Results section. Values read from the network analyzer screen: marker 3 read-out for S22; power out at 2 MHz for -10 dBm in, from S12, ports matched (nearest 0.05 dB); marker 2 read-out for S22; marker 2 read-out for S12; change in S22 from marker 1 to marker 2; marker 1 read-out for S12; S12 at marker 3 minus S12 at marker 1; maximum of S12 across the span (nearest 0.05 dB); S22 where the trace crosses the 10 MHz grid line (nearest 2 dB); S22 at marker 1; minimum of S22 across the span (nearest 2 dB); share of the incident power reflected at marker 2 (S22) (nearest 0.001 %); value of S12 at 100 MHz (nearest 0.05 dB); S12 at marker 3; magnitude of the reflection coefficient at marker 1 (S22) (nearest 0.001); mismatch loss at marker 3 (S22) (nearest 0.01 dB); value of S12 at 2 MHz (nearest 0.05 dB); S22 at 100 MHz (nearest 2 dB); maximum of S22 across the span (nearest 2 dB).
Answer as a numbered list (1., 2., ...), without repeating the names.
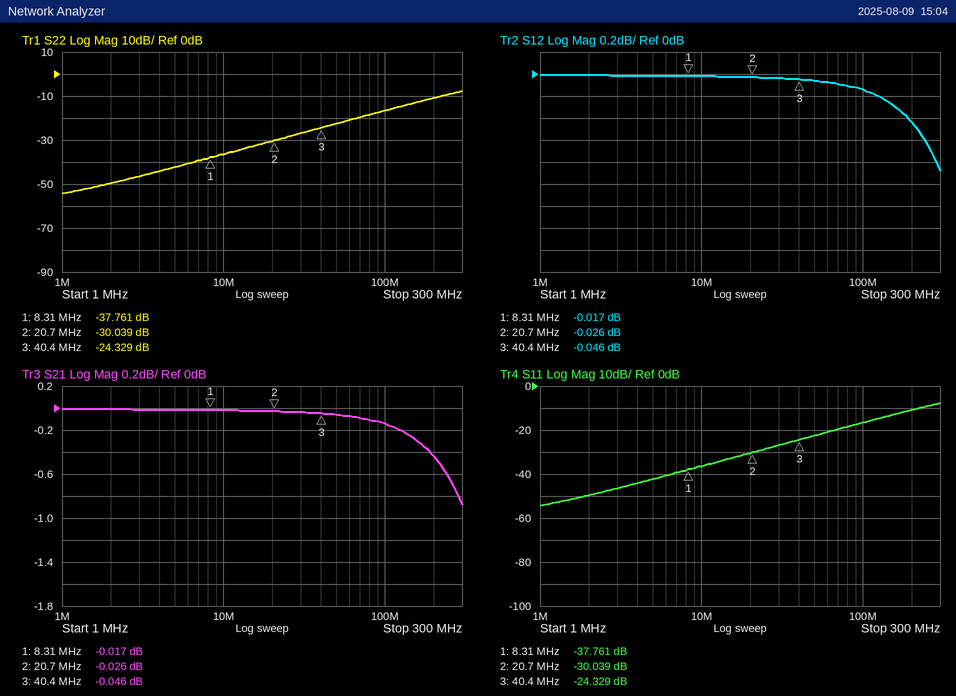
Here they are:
1. -24.329 dB
2. -10.00 dBm
3. -30.039 dB
4. -0.026 dB
5. 7.722 dB
6. -0.017 dB
7. -0.029 dB
8. 0.00 dB
9. -36 dB
10. -37.761 dB
11. -54 dB
12. 0.099 %
13. -0.15 dB
14. -0.046 dB
15. 0.013
16. 0.02 dB
17. 0.00 dB
18. -16 dB
19. -8 dB
